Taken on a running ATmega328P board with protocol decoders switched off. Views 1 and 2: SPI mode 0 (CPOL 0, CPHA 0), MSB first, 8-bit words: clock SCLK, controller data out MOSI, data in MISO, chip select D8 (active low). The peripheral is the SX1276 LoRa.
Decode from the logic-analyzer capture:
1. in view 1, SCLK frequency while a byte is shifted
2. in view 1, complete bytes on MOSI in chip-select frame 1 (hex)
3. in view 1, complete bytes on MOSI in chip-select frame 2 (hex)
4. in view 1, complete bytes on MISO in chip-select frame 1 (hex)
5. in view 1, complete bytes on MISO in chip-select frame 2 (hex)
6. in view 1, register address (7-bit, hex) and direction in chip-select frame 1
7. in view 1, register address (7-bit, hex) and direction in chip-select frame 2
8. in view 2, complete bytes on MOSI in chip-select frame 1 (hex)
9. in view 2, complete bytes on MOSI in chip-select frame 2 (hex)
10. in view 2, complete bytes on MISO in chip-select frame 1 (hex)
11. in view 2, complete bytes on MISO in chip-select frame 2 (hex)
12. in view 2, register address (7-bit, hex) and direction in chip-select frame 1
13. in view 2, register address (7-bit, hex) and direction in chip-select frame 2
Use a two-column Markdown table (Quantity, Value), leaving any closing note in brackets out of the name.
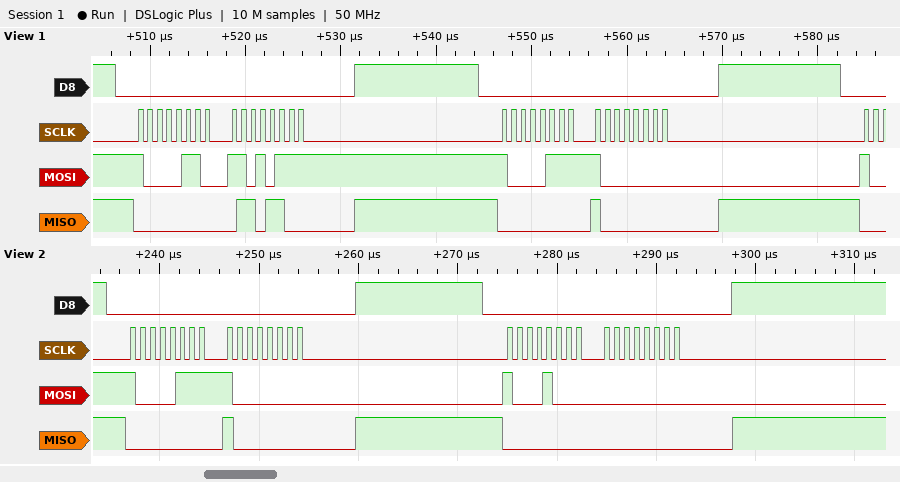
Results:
| Quantity | Value |
|---|---|
| in view 1, SCLK frequency while a byte is shifted | 1 MHz |
| in view 1, complete bytes on MOSI in chip-select frame 1 | 0x86 0xD7 |
| in view 1, complete bytes on MOSI in chip-select frame 2 | 0x87 0x80 |
| in view 1, complete bytes on MISO in chip-select frame 1 | 0x00 0x6C |
| in view 1, complete bytes on MISO in chip-select frame 2 | 0x00 0x80 |
| in view 1, register address (7-bit, hex) and direction in chip-select frame 1 | 0x06 write |
| in view 1, register address (7-bit, hex) and direction in chip-select frame 2 | 0x07 write |
| in view 2, complete bytes on MOSI in chip-select frame 1 | 87 80 |
| in view 2, complete bytes on MOSI in chip-select frame 2 | 88 00 |
| in view 2, complete bytes on MISO in chip-select frame 1 | 00 80 |
| in view 2, complete bytes on MISO in chip-select frame 2 | 00 00 |
| in view 2, register address (7-bit, hex) and direction in chip-select frame 1 | 0x07 write |
| in view 2, register address (7-bit, hex) and direction in chip-select frame 2 | 0x08 write |
